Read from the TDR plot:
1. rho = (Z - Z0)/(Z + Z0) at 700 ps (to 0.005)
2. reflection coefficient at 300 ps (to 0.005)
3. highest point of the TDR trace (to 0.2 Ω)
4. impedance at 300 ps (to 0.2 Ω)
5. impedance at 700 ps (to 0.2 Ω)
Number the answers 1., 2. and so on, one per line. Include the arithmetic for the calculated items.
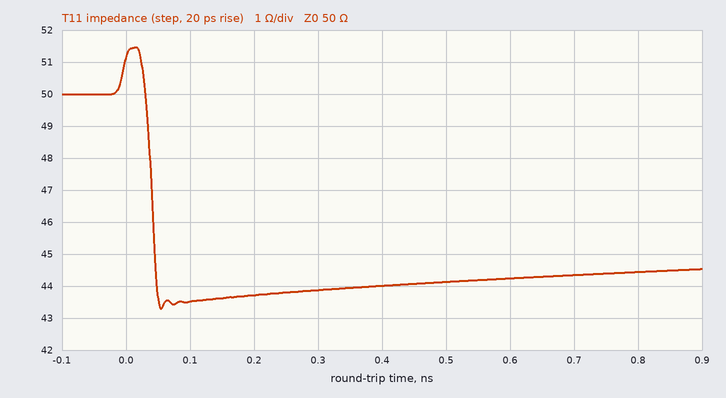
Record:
1. (44.4 − 50)/(44.4 + 50) ≈ -0.0593, so -0.060 to the nearest 0.005
2. (43.8 − 50)/(43.8 + 50) ≈ -0.0661, so -0.065 to the nearest 0.005
3. 51.4 Ω
4. 43.8 Ω
5. 44.4 Ω
